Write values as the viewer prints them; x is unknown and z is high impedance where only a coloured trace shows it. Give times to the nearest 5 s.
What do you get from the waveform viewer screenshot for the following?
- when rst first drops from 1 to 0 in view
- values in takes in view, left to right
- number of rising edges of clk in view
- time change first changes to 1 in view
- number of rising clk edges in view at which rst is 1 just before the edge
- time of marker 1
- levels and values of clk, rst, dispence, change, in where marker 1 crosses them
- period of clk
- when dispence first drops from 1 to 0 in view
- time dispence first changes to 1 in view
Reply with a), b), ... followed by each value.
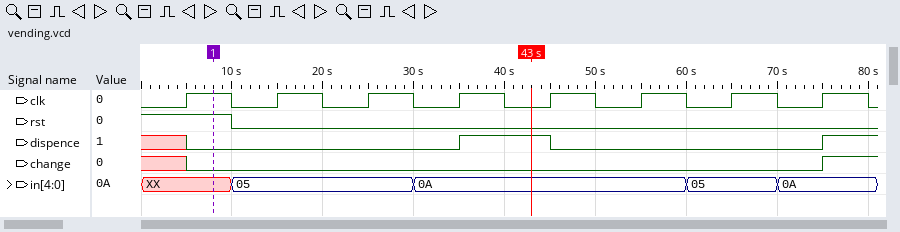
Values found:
a) 10 s
b) XX, 05, 0A, 05, 0A
c) 8
d) 75 s
e) 1
f) 10 s
g) clk=1, rst=1, dispence=0, change=0, in=XX
h) 10 s
i) 45 s
j) 35 s
